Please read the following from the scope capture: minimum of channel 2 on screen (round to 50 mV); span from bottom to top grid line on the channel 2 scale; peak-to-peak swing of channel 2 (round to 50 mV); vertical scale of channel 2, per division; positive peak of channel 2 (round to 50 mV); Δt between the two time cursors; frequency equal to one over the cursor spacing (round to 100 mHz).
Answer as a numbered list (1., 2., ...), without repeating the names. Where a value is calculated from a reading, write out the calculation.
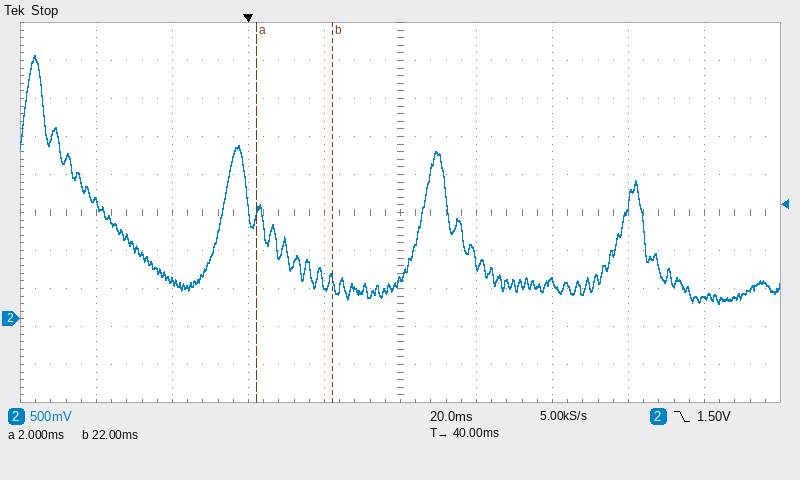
1. 200 mV
2. 5 V
3. 3.45 V − (200 mV) = 3.25 V
4. 500 mV
5. 3.45 V
6. 22 ms − (2 ms) = 20 ms
7. 1 / 20 ms ≈ 50.0 Hz
